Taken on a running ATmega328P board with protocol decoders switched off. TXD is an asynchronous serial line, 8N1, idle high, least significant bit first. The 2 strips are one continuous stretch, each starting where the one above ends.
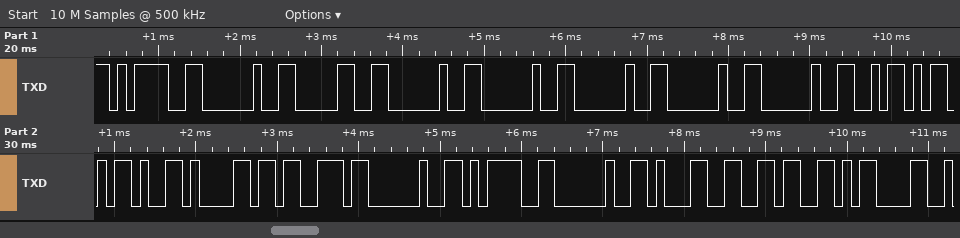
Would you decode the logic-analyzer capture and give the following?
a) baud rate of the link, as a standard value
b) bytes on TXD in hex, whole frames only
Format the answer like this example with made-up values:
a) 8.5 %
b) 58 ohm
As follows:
a) 9600 baud
b) 0x3D 0x20 0x30 0x20 0x20 0x20 0x20 0x20 0x5A 0x2D 0x61 0x73 0x20 0x3D 0x20 0x31 0x36 0x0D
